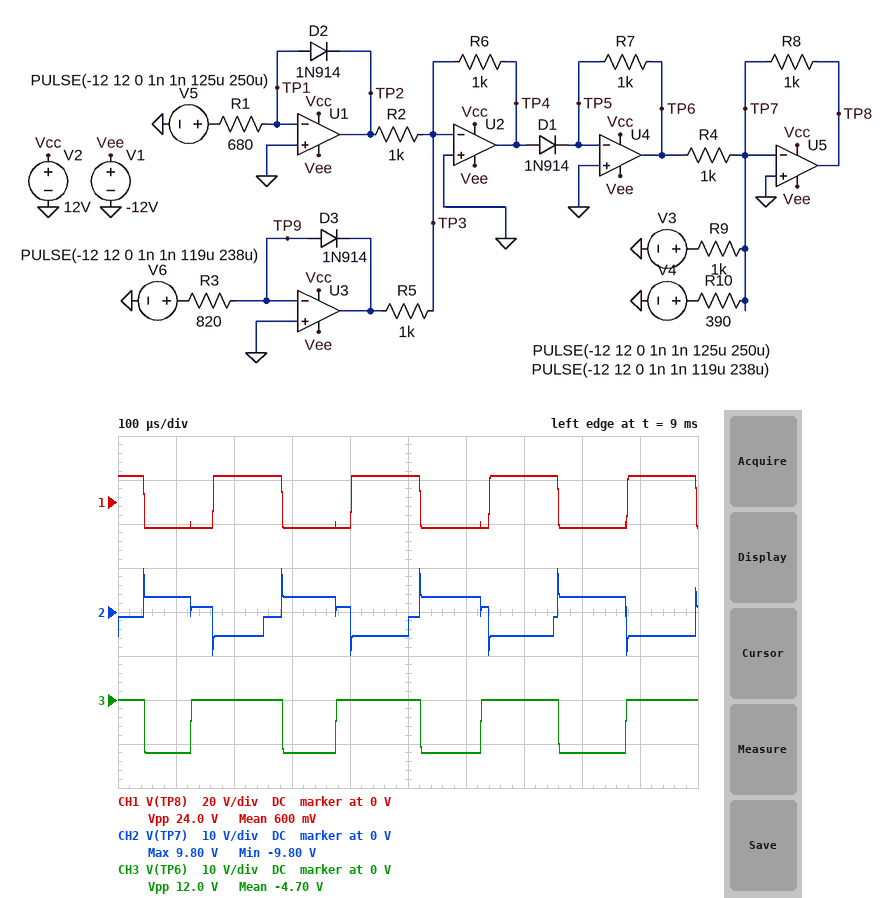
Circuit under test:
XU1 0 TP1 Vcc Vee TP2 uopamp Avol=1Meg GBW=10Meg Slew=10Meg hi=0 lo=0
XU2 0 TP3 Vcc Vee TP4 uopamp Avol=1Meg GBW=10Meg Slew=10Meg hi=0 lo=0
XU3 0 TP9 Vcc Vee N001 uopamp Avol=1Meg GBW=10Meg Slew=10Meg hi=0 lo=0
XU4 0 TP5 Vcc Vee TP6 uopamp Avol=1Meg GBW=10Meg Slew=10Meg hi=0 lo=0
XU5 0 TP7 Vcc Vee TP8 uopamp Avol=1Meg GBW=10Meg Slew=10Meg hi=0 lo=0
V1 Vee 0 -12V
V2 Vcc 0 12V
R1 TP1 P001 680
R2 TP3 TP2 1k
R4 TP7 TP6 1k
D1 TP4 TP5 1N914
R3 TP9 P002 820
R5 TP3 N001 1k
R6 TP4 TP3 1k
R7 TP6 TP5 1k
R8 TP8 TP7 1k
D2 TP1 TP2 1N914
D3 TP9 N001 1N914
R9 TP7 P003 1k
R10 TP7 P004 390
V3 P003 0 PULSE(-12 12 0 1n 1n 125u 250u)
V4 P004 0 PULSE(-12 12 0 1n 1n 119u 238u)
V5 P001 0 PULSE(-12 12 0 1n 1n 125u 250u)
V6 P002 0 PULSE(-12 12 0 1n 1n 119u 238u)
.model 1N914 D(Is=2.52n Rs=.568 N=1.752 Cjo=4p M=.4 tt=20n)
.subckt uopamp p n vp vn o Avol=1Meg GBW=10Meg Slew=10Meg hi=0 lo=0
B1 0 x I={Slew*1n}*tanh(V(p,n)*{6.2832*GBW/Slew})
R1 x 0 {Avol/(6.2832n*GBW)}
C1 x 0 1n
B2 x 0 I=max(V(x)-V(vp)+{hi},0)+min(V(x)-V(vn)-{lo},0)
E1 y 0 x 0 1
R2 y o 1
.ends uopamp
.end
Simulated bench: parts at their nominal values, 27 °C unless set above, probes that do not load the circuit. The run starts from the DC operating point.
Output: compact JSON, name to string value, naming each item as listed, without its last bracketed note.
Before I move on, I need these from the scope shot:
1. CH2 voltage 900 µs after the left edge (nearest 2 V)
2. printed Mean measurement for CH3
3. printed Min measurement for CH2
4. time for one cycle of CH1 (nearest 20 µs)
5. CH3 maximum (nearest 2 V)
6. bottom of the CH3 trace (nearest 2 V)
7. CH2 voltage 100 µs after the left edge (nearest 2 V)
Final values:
{"CH2 voltage 900 µs after the left edge": "-6 V", "printed Mean measurement for CH3": "-4.70 V", "printed Min measurement for CH2": "-9.80 V", "time for one cycle of CH1": "240 µs", "CH3 maximum": "0 V", "bottom of the CH3 trace": "-12 V", "CH2 voltage 100 µs after the left edge": "4 V"}
